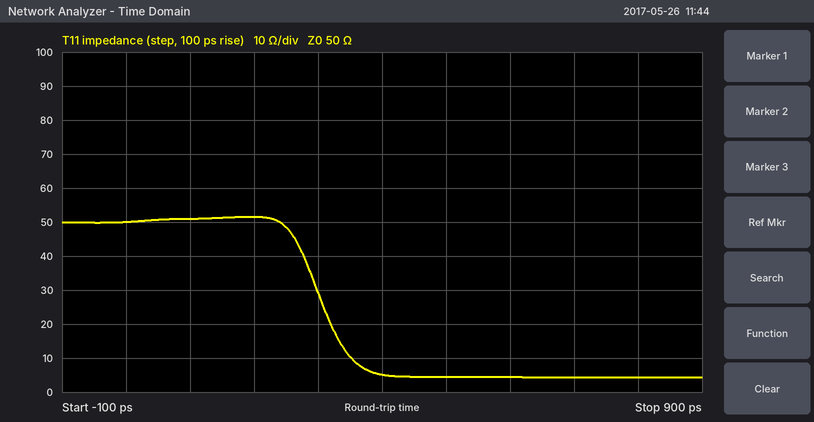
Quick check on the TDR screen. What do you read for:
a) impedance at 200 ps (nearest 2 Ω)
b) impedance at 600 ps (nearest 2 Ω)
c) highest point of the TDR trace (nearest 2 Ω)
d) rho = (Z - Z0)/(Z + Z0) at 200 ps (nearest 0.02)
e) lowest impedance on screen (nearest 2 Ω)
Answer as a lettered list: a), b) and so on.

a) 52 Ω
b) 4 Ω
c) 52 Ω
d) +0.02
e) 4 Ω
